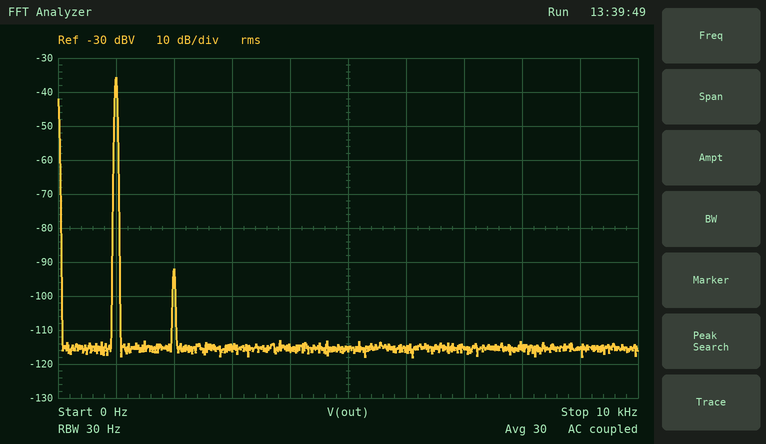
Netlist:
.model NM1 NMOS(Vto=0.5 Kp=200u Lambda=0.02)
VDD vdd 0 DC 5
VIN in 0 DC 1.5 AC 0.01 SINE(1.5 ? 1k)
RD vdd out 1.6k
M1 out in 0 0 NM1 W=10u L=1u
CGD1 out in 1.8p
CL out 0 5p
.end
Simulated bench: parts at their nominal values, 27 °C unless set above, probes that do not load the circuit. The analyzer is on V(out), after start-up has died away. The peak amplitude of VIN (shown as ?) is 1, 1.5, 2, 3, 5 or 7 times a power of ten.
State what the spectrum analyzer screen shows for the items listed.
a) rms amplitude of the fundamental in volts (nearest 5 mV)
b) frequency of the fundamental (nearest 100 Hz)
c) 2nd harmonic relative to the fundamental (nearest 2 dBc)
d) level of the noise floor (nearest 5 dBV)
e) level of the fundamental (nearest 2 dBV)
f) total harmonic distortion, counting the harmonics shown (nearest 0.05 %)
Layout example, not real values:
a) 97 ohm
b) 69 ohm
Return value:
a) 15 mV
b) 1.0 kHz
c) -56 dBc
d) -115 dBV
e) -36 dBV
f) 0.15 %
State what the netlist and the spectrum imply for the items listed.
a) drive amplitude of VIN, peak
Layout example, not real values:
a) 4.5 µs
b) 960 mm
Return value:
a) 7 mV
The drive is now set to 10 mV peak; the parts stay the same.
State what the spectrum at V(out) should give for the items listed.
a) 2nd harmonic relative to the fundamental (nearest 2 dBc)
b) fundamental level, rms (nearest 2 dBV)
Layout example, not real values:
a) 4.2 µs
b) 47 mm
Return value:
a) -54 dBc
b) -32 dBV
